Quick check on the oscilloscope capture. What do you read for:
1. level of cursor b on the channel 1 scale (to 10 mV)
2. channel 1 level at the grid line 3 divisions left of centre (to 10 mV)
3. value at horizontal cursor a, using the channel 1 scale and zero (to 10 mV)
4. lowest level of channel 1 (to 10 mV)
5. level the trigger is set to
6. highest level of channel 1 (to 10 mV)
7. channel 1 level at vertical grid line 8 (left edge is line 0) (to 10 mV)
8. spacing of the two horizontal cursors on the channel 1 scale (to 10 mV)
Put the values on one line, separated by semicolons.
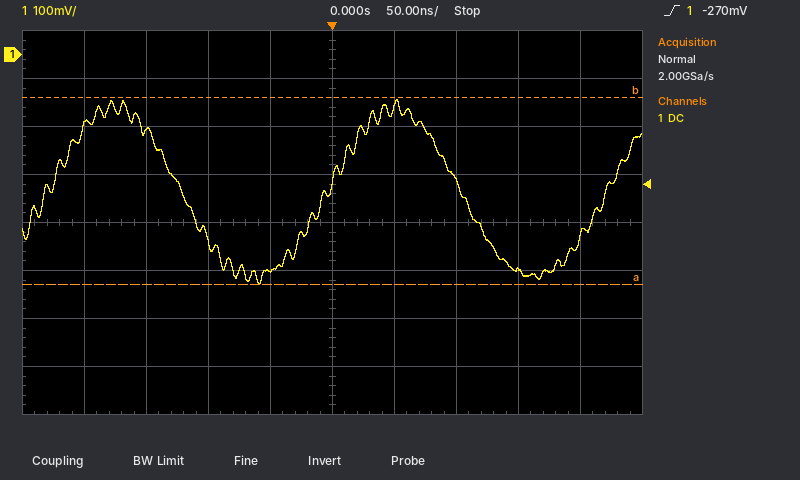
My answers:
-90 mV; -160 mV; -480 mV; -480 mV; -270 mV; -90 mV; -450 mV; 390 mV
